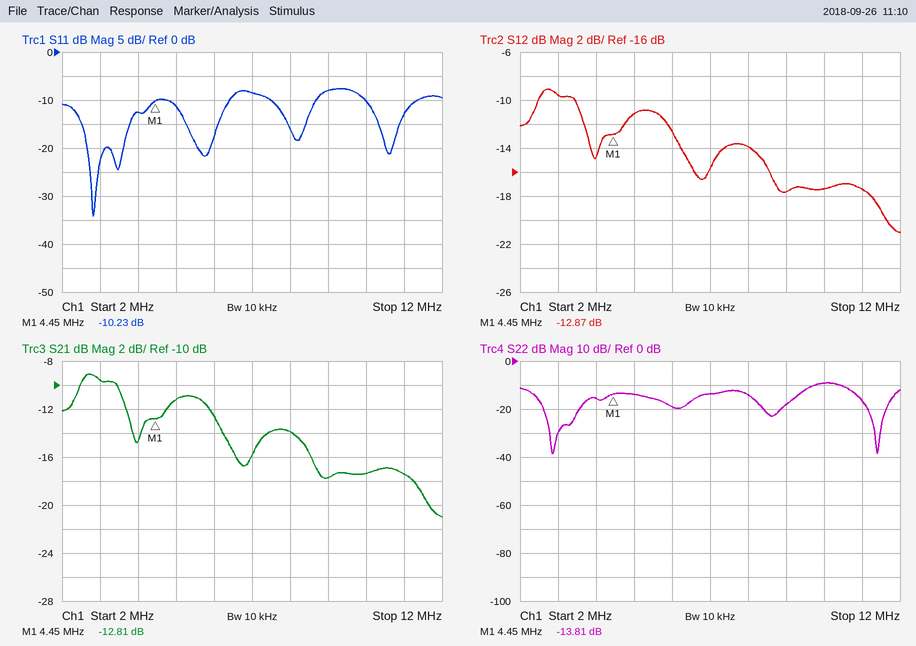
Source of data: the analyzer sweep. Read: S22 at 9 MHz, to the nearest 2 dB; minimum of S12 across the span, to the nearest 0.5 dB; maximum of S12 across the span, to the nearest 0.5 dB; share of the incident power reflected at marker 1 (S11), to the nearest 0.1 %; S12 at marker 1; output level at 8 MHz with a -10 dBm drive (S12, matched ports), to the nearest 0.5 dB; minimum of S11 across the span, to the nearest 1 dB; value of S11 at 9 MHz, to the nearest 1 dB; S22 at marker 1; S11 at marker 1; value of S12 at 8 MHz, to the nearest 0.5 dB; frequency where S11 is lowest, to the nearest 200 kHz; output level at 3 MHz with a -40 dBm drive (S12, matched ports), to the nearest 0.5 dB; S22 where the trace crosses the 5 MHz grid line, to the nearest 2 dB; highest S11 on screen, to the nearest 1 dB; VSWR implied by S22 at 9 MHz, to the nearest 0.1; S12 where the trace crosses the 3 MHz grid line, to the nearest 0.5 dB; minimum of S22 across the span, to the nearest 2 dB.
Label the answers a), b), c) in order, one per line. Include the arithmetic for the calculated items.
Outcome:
a) -18 dB
b) -21.0 dB
c) -9.0 dB
d) 10^(-10.23/10) ≈ 9.5 %
e) -12.87 dB
f) -10 dBm + (-14.0 dB) = -24.0 dBm
g) -34 dB
h) -8 dB
i) -13.81 dB
j) -10.23 dB
k) -14.0 dB
l) 2.8 MHz
m) -40 dBm + (-9.5 dB) = -49.5 dBm
n) -14 dB
o) -8 dB
p) |Γ| = 10^(-18/20) = 0.1259; VSWR = (1 + 0.1259)/(1 − 0.1259) ≈ 1.3
q) -9.5 dB
r) -38 dB
